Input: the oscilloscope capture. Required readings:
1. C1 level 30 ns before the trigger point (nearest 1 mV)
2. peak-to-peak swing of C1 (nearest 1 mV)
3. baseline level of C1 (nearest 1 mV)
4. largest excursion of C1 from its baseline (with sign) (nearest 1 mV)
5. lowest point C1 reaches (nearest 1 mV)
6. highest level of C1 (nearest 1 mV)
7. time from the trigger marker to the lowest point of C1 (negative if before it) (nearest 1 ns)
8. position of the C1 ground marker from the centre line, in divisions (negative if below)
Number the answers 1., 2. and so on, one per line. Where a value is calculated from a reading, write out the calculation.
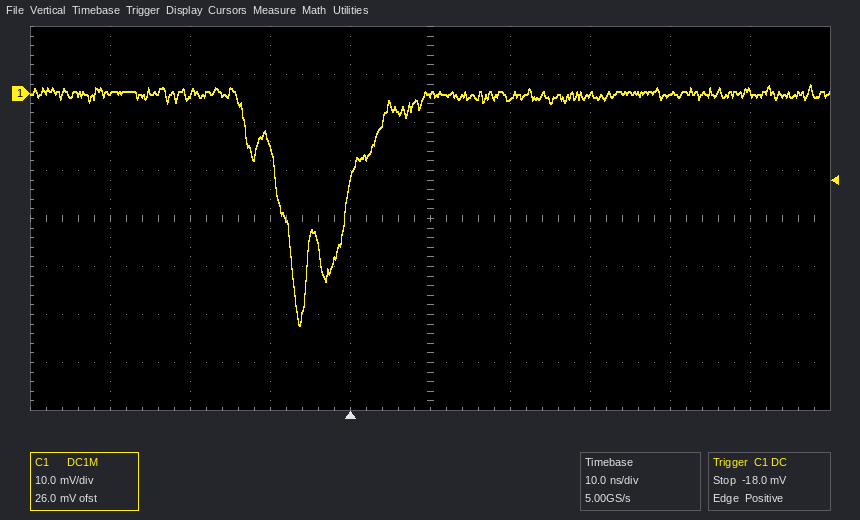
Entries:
1. 0 mV
2. 2 mV − (-48 mV) = 50 mV
3. 0 mV
4. -48 mV − (0 mV) = -48 mV
5. -48 mV
6. 2 mV
7. -6 ns
8. +2.6 div
